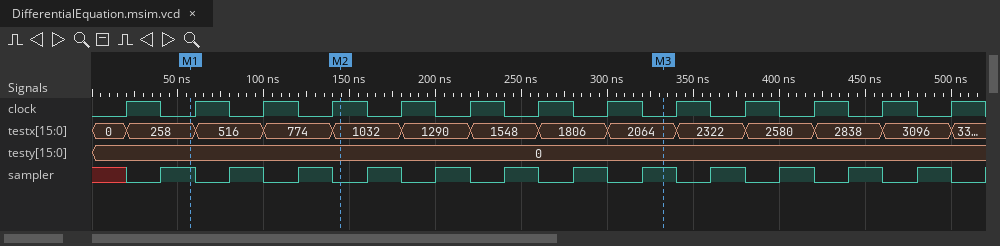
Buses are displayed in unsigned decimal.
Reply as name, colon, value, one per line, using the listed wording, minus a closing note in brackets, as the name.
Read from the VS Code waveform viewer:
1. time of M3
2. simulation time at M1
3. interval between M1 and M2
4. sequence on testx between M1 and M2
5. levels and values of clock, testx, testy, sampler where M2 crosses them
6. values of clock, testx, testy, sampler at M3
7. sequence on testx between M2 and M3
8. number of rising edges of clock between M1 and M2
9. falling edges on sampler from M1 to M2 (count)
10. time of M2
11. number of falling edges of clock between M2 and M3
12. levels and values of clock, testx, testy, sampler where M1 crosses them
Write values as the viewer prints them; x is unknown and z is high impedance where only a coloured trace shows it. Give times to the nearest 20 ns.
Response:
time of M3: 340 ns
simulation time at M1: 60 ns
interval between M1 and M2: 80 ns
sequence on testx between M1 and M2: 258, 516, 774, 1032
levels and values of clock, testx, testy, sampler where M2 crosses them: clock=1, testx=1032, testy=0, sampler=0
values of clock, testx, testy, sampler at M3: clock=0, testx=2064, testy=0, sampler=1
sequence on testx between M2 and M3: 1032, 1290, 1548, 1806, 2064
number of rising edges of clock between M1 and M2: 3
falling edges on sampler from M1 to M2: 3
time of M2: 140 ns
number of falling edges of clock between M2 and M3: 5
levels and values of clock, testx, testy, sampler where M1 crosses them: clock=0, testx=258, testy=0, sampler=1
